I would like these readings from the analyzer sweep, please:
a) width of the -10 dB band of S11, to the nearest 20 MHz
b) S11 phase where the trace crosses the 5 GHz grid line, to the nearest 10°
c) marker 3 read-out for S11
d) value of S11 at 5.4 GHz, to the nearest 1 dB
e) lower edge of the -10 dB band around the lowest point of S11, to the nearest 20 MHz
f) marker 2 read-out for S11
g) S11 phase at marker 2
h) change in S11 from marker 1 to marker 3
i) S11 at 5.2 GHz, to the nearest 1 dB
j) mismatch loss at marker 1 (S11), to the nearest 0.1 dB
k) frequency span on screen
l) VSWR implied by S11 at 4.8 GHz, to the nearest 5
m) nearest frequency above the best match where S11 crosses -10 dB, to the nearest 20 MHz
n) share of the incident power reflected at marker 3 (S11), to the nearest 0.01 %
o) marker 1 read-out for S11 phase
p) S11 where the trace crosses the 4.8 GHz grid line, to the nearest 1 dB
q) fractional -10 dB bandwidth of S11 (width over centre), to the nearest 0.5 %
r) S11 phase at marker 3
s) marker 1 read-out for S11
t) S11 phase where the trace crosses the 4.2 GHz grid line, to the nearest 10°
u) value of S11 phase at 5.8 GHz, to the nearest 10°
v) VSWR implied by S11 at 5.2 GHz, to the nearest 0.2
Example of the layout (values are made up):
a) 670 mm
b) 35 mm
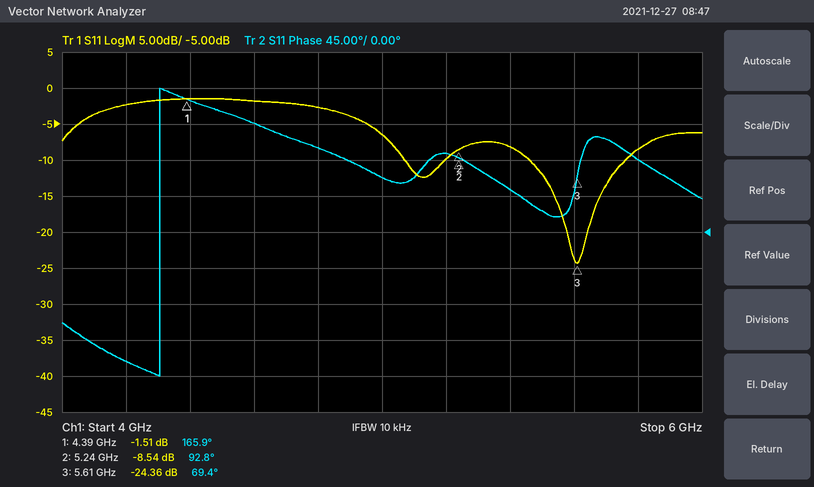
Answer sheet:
a) 300 MHz
b) 70°
c) -24.36 dB
d) -8 dB
e) 5.46 GHz
f) -8.54 dB
g) 92.8°
h) -22.85 dB
i) -10 dB
j) 5.3 dB
k) 2 GHz
l) 5
m) 5.76 GHz
n) 0.37 %
o) 165.9°
p) -3 dB
q) 5.5 %
r) 69.4°
s) -1.51 dB
t) -160°
u) 90°
v) 2.0
